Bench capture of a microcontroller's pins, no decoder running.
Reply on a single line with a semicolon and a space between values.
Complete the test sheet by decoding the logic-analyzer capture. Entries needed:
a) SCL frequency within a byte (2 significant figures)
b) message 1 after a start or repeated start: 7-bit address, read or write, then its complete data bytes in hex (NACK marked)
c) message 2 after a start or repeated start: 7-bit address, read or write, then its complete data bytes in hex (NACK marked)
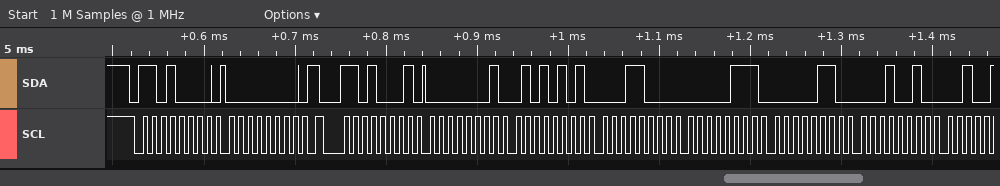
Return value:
100 kHz; 0x68 write: 00; 0x68 read: 01 55 18 07 06 12
